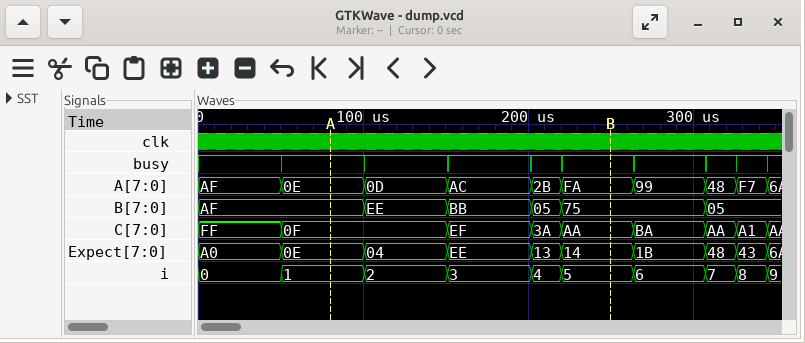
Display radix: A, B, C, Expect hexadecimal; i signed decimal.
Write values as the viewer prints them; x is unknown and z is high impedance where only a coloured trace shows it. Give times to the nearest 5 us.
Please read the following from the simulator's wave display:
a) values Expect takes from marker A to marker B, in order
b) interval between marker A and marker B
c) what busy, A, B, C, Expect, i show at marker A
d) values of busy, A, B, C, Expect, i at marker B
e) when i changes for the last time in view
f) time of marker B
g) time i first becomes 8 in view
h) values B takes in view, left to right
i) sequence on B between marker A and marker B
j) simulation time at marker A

0E, 04, EE, 13, 14
170 us
busy=1, A=0E, B=AF, C=0F, Expect=0E, i=1
busy=1, A=FA, B=75, C=AA, Expect=14, i=5
345 us
250 us
325 us
AF, EE, BB, 05, 75, 05
AF, EE, BB, 05, 75
80 us
